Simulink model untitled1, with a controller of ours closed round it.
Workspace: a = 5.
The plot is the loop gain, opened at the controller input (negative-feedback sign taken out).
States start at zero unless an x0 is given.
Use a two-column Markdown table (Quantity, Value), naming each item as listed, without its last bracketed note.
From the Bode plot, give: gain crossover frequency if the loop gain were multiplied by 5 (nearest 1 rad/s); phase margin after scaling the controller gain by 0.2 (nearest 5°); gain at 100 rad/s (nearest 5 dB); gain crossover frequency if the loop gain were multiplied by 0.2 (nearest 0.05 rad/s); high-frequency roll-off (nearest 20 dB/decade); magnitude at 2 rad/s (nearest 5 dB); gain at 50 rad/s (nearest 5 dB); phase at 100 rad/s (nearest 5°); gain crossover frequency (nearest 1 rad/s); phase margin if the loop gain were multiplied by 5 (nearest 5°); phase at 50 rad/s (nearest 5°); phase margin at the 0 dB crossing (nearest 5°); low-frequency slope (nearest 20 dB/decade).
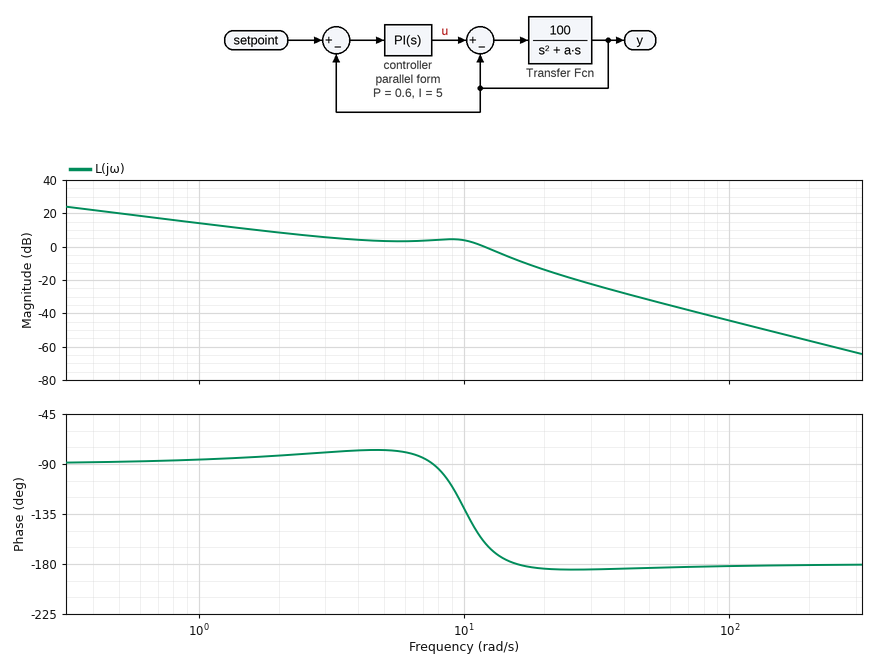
| Quantity | Value |
|---|---|
| gain crossover frequency if the loop gain were multiplied by 5 | 20 rad/s |
| phase margin after scaling the controller gain by 0.2 | 95° |
| gain at 100 rad/s | -45 dB |
| gain crossover frequency if the loop gain were multiplied by 0.2 | 1.00 rad/s |
| high-frequency roll-off | -40 dB/decade |
| magnitude at 2 rad/s | 10 dB |
| gain at 50 rad/s | -30 dB |
| phase at 100 rad/s | -180° |
| gain crossover frequency | 12 rad/s |
| phase margin if the loop gain were multiplied by 5 | -5° |
| phase at 50 rad/s | -185° |
| phase margin at the 0 dB crossing | 20° |
| low-frequency slope | -20 dB/decade |
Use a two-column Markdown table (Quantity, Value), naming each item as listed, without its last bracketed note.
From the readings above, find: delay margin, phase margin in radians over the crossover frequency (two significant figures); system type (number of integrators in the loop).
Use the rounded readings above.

| Quantity | Value |
|---|---|
| delay margin, phase margin in radians over the crossover frequency | 0.029 s |
| system type | 1 |
